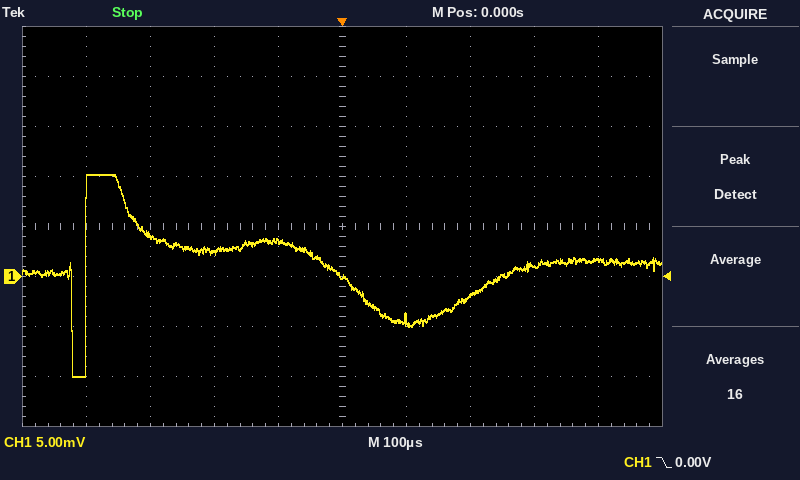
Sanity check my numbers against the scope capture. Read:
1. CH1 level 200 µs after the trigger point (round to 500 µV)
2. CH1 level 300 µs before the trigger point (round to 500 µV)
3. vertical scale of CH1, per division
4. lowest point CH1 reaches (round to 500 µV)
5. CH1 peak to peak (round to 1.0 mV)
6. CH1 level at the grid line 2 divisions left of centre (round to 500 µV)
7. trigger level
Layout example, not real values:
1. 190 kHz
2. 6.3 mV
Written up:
1. -2.0 mV
2. 4.0 mV
3. 5 mV
4. -10.0 mV
5. 20.0 mV
6. 2.5 mV
7. 0.00 V
